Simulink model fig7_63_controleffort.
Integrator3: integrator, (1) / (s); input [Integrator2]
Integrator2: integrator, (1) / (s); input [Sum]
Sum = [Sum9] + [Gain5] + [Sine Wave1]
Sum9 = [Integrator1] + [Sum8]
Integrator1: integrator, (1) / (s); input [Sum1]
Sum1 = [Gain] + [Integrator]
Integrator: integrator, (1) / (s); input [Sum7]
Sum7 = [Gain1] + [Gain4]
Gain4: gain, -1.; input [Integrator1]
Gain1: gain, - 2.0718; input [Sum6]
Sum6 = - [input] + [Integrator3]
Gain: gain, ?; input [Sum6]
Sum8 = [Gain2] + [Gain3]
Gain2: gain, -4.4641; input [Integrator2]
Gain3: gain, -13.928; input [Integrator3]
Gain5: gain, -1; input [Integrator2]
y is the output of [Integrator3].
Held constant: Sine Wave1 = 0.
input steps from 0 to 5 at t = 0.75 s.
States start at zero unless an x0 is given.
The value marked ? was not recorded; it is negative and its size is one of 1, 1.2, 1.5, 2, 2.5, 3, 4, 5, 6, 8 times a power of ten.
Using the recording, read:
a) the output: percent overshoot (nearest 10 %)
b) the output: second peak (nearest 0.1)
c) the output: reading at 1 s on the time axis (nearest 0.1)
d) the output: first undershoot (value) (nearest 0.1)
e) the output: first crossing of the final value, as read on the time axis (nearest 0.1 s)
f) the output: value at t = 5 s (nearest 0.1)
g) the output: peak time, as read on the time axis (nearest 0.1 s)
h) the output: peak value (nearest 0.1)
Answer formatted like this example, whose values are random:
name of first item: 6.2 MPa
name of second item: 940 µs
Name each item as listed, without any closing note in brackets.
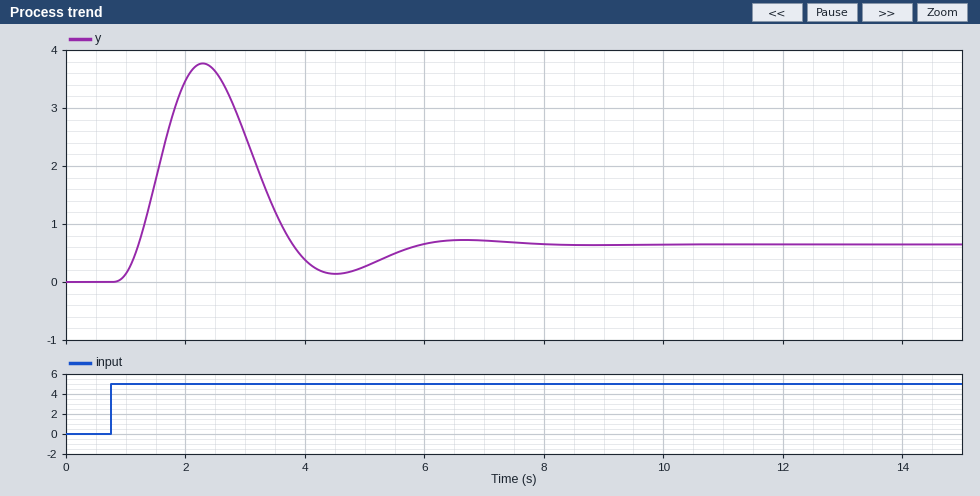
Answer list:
the output: percent overshoot: 480 %
the output: second peak: 0.7
the output: reading at 1 s on the time axis: 0.1
the output: first undershoot (value): 0.1
the output: first crossing of the final value, as read on the time axis: 1.2 s
the output: value at t = 5 s: 0.3
the output: peak time, as read on the time axis: 2.3 s
the output: peak value: 3.8
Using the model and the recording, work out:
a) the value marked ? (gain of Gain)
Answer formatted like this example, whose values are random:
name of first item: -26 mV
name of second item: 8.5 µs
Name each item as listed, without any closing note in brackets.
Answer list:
the value marked ?: -15
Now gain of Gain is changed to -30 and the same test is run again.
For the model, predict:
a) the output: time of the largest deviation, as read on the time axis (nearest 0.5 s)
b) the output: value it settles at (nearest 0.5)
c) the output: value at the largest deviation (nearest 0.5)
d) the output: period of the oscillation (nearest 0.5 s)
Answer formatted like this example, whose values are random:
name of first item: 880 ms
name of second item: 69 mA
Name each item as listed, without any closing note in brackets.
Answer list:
the output: time of the largest deviation, as read on the time axis: 2.0 s
the output: value it settles at: 0.5
the output: value at the largest deviation: 5.5
the output: period of the oscillation: 2.5 s
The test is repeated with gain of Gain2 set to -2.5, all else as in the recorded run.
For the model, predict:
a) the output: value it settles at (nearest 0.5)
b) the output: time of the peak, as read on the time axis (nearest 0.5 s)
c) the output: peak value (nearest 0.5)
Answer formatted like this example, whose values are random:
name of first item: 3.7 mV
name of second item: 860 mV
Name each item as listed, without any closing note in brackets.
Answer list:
the output: value it settles at: 0.5
the output: time of the peak, as read on the time axis: 2.0 s
the output: peak value: 4.0
